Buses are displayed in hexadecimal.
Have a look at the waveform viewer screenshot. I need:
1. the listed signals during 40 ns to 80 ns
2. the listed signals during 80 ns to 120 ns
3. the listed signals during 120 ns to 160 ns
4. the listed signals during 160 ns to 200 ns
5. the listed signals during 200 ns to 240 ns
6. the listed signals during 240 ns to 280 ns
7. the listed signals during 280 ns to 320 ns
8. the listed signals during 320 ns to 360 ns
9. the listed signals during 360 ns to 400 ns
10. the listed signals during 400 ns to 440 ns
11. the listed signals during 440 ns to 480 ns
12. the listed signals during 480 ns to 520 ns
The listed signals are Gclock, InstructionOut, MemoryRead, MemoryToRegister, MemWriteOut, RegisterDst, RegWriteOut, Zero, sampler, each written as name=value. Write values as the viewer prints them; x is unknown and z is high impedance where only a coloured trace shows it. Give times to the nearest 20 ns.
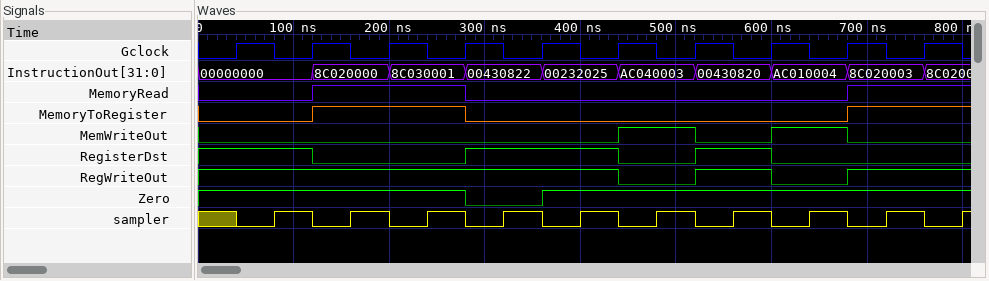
Gclock=1, InstructionOut=00000000, MemoryRead=0, MemoryToRegister=0, MemWriteOut=0, RegisterDst=1, RegWriteOut=1, Zero=1, sampler=0
Gclock=0, InstructionOut=00000000, MemoryRead=0, MemoryToRegister=0, MemWriteOut=0, RegisterDst=1, RegWriteOut=1, Zero=1, sampler=1
Gclock=1, InstructionOut=8C020000, MemoryRead=1, MemoryToRegister=1, MemWriteOut=0, RegisterDst=0, RegWriteOut=1, Zero=1, sampler=0
Gclock=0, InstructionOut=8C020000, MemoryRead=1, MemoryToRegister=1, MemWriteOut=0, RegisterDst=0, RegWriteOut=1, Zero=1, sampler=1
Gclock=1, InstructionOut=8C030001, MemoryRead=1, MemoryToRegister=1, MemWriteOut=0, RegisterDst=0, RegWriteOut=1, Zero=1, sampler=0
Gclock=0, InstructionOut=8C030001, MemoryRead=1, MemoryToRegister=1, MemWriteOut=0, RegisterDst=0, RegWriteOut=1, Zero=1, sampler=1
Gclock=1, InstructionOut=00430822, MemoryRead=0, MemoryToRegister=0, MemWriteOut=0, RegisterDst=1, RegWriteOut=1, Zero=0, sampler=0
Gclock=0, InstructionOut=00430822, MemoryRead=0, MemoryToRegister=0, MemWriteOut=0, RegisterDst=1, RegWriteOut=1, Zero=0, sampler=1
Gclock=1, InstructionOut=00232025, MemoryRead=0, MemoryToRegister=0, MemWriteOut=0, RegisterDst=1, RegWriteOut=1, Zero=1, sampler=0
Gclock=0, InstructionOut=00232025, MemoryRead=0, MemoryToRegister=0, MemWriteOut=0, RegisterDst=1, RegWriteOut=1, Zero=1, sampler=1
Gclock=1, InstructionOut=AC040003, MemoryRead=0, MemoryToRegister=0, MemWriteOut=1, RegisterDst=0, RegWriteOut=0, Zero=1, sampler=0
Gclock=0, InstructionOut=AC040003, MemoryRead=0, MemoryToRegister=0, MemWriteOut=1, RegisterDst=0, RegWriteOut=0, Zero=1, sampler=1
